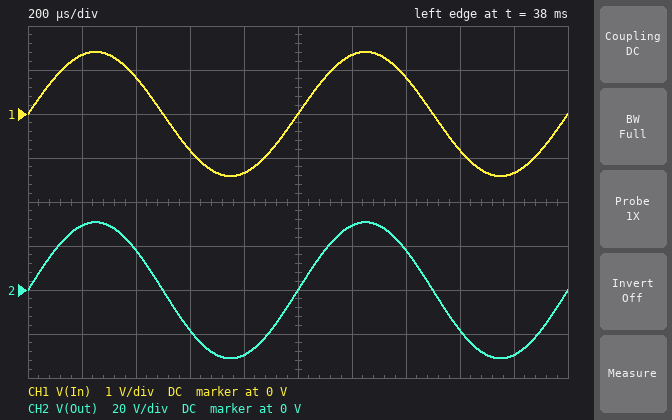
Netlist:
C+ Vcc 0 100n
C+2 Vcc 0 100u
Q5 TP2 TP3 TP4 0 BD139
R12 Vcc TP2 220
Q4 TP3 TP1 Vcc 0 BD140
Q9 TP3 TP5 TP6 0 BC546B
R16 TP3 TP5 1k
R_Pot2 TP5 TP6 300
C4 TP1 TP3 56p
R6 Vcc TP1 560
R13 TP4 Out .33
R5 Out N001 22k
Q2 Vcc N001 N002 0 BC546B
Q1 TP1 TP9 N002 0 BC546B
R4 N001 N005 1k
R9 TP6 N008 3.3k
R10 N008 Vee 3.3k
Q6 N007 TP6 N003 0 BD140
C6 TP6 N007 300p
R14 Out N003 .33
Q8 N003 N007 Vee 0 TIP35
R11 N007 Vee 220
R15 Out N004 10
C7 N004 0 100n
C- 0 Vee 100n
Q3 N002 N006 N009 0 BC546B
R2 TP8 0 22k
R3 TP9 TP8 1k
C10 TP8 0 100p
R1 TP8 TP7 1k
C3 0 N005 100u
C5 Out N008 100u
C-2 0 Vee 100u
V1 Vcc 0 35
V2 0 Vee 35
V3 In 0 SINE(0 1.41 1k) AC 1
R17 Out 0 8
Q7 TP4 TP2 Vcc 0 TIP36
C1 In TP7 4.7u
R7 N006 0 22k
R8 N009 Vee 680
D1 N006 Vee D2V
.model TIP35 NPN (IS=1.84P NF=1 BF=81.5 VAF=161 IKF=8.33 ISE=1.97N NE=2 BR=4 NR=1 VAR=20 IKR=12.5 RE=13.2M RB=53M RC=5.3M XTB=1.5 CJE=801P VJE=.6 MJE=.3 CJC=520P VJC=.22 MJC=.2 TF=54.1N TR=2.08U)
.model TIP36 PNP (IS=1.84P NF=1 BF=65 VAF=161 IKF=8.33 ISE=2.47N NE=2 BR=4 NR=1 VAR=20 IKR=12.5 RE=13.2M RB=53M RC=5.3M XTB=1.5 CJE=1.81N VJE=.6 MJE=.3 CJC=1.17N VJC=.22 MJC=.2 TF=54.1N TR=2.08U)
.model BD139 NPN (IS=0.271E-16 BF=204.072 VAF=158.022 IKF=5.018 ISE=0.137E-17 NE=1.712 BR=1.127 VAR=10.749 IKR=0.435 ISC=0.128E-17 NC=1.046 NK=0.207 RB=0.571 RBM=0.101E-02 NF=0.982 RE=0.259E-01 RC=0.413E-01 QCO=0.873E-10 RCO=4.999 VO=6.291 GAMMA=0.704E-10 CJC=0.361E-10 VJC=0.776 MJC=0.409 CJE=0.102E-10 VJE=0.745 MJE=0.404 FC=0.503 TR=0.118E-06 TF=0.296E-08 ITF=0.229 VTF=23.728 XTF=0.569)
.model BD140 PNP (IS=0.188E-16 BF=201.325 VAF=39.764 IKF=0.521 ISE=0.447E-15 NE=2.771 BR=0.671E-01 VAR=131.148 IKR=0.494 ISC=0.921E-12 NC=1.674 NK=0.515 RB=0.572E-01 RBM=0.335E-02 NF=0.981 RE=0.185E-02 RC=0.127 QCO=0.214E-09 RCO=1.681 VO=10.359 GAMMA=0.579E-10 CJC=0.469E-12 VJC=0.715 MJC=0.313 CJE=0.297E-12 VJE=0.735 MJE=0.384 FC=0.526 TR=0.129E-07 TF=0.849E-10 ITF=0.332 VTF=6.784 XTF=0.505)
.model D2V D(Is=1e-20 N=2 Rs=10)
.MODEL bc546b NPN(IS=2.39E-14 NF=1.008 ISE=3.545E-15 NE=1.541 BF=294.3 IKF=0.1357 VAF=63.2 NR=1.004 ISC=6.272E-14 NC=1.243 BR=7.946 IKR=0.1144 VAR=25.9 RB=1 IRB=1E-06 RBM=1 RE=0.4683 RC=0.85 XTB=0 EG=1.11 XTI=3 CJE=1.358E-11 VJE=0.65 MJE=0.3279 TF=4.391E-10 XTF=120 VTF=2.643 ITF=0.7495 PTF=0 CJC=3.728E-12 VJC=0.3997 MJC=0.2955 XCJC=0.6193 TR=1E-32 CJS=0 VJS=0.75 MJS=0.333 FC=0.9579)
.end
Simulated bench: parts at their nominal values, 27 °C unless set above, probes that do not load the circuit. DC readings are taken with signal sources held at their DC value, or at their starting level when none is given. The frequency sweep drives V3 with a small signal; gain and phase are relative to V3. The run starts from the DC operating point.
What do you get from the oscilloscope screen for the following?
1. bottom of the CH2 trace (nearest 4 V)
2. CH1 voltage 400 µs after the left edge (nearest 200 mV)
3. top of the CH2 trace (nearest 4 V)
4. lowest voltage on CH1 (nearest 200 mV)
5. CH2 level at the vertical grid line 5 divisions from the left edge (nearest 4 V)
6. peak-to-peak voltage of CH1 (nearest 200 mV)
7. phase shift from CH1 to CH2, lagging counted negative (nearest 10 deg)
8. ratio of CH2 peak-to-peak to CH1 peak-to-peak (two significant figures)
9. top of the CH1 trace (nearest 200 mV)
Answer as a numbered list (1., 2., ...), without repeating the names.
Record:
1. -32 V
2. 800 mV
3. 32 V
4. -1.4 V
5. 0 V
6. 2.8 V
7. 0 deg
8. 22
9. 1.4 V
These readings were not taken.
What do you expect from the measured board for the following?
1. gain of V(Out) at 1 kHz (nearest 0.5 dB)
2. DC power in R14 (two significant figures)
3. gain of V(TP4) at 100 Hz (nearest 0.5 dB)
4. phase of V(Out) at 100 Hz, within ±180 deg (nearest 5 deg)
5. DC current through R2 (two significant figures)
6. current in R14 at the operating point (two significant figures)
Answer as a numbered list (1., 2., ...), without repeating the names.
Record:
1. 27.0 dB
2. 1.0 W
3. 27.0 dB
4. 0 deg
5. 3.4 µA
6. 1.7 A
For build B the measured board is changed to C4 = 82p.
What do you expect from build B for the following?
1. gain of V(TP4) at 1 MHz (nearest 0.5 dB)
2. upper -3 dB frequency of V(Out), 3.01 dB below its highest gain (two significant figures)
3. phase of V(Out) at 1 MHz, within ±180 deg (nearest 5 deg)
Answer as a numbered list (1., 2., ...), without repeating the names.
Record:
1. 25.0 dB
2. 1.2 MHz
3. -90 deg
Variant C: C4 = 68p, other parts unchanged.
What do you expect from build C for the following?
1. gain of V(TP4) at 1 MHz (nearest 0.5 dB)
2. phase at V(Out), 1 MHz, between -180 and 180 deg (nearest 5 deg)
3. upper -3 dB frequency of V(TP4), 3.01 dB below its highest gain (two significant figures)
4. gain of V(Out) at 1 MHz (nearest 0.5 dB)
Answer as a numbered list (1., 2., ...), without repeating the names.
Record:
1. 26.0 dB
2. -80 deg
3. 1.4 MHz
4. 25.5 dB
